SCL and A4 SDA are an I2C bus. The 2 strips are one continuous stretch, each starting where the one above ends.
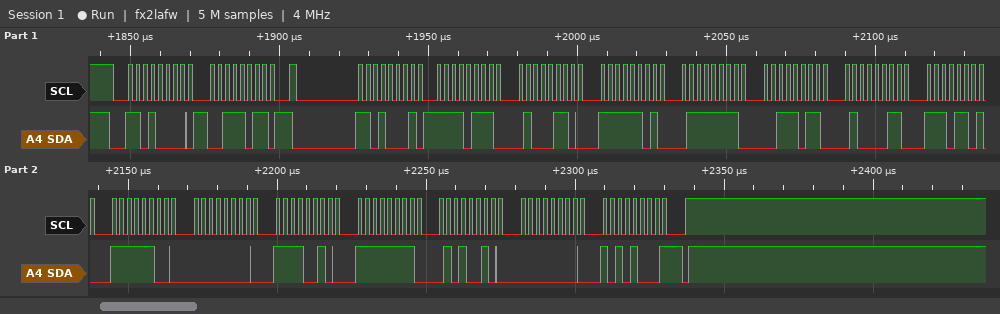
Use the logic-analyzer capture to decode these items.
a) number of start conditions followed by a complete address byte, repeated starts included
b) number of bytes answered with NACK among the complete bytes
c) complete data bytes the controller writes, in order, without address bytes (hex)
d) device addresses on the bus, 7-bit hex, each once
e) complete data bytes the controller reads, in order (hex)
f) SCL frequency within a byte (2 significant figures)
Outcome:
2
1
3B
0x68
F7 46 FD 7F 3B 43 ED FC 00 F2 FF 52 00 A8
400 kHz
